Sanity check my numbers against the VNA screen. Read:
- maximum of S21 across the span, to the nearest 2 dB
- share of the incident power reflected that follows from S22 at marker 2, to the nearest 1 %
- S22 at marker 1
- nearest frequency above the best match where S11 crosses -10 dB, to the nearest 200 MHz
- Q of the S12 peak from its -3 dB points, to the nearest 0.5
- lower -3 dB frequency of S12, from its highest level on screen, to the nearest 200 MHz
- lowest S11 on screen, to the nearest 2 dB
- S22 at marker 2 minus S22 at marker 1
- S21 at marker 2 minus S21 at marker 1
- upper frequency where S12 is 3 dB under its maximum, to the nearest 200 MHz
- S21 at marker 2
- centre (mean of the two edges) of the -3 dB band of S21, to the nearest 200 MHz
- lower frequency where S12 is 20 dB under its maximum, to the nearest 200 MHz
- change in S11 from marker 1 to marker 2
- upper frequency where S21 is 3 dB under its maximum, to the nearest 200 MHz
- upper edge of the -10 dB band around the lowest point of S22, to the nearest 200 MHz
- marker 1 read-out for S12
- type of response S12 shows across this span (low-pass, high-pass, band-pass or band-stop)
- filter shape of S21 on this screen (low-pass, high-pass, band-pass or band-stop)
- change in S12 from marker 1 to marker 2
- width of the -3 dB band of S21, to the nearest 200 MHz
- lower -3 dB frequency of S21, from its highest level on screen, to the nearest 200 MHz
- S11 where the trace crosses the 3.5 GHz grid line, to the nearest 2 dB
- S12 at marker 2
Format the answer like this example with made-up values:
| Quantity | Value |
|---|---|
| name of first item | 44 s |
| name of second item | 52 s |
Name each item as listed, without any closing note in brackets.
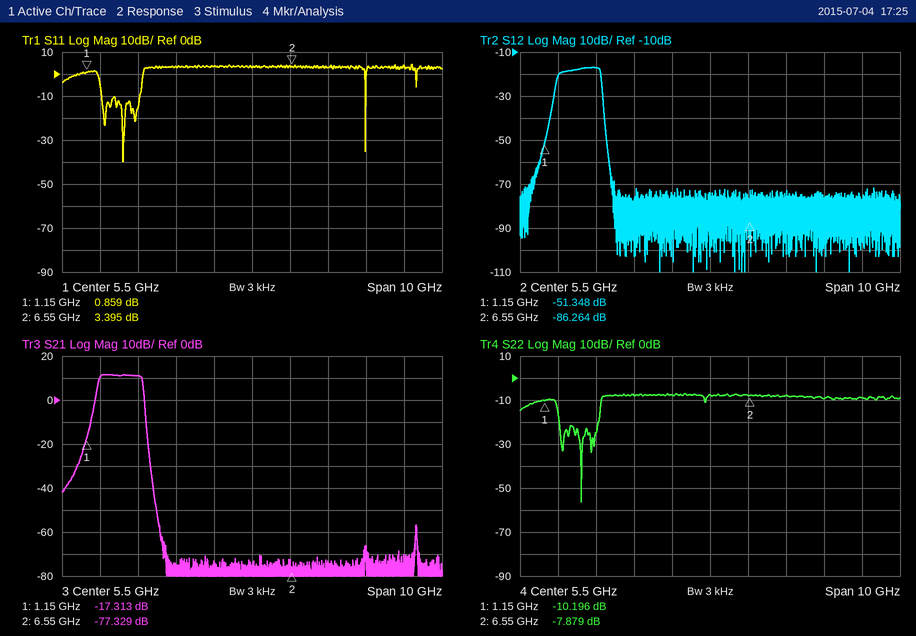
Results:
| Quantity | Value |
|---|---|
| maximum of S21 across the span, to the nearest 2 dB | 12 dB |
| share of the incident power reflected that follows from S22 at marker 2, to the nearest 1 % | 16 % |
| S22 at marker 1 | -10.196 dB |
| nearest frequency above the best match where S11 crosses -10 dB, to the nearest 200 MHz | 2.6 GHz |
| Q of the S12 peak from its -3 dB points, to the nearest 0.5 | 2.0 |
| lower -3 dB frequency of S12, from its highest level on screen, to the nearest 200 MHz | 1.6 GHz |
| lowest S11 on screen, to the nearest 2 dB | -40 dB |
| S22 at marker 2 minus S22 at marker 1 | 2.317 dB |
| S21 at marker 2 minus S21 at marker 1 | -60.016 dB |
| upper frequency where S12 is 3 dB under its maximum, to the nearest 200 MHz | 2.6 GHz |
| S21 at marker 2 | -77.329 dB |
| centre (mean of the two edges) of the -3 dB band of S21, to the nearest 200 MHz | 2.0 GHz |
| lower frequency where S12 is 20 dB under its maximum, to the nearest 200 MHz | 1.4 GHz |
| change in S11 from marker 1 to marker 2 | 2.536 dB |
| upper frequency where S21 is 3 dB under its maximum, to the nearest 200 MHz | 2.6 GHz |
| upper edge of the -10 dB band around the lowest point of S22, to the nearest 200 MHz | 2.6 GHz |
| marker 1 read-out for S12 | -51.348 dB |
| type of response S12 shows across this span | band-pass |
| filter shape of S21 on this screen | band-pass |
| change in S12 from marker 1 to marker 2 | -34.916 dB |
| width of the -3 dB band of S21, to the nearest 200 MHz | 1.2 GHz |
| lower -3 dB frequency of S21, from its highest level on screen, to the nearest 200 MHz | 1.4 GHz |
| S11 where the trace crosses the 3.5 GHz grid line, to the nearest 2 dB | 4 dB |
| S12 at marker 2 | -86.264 dB |
